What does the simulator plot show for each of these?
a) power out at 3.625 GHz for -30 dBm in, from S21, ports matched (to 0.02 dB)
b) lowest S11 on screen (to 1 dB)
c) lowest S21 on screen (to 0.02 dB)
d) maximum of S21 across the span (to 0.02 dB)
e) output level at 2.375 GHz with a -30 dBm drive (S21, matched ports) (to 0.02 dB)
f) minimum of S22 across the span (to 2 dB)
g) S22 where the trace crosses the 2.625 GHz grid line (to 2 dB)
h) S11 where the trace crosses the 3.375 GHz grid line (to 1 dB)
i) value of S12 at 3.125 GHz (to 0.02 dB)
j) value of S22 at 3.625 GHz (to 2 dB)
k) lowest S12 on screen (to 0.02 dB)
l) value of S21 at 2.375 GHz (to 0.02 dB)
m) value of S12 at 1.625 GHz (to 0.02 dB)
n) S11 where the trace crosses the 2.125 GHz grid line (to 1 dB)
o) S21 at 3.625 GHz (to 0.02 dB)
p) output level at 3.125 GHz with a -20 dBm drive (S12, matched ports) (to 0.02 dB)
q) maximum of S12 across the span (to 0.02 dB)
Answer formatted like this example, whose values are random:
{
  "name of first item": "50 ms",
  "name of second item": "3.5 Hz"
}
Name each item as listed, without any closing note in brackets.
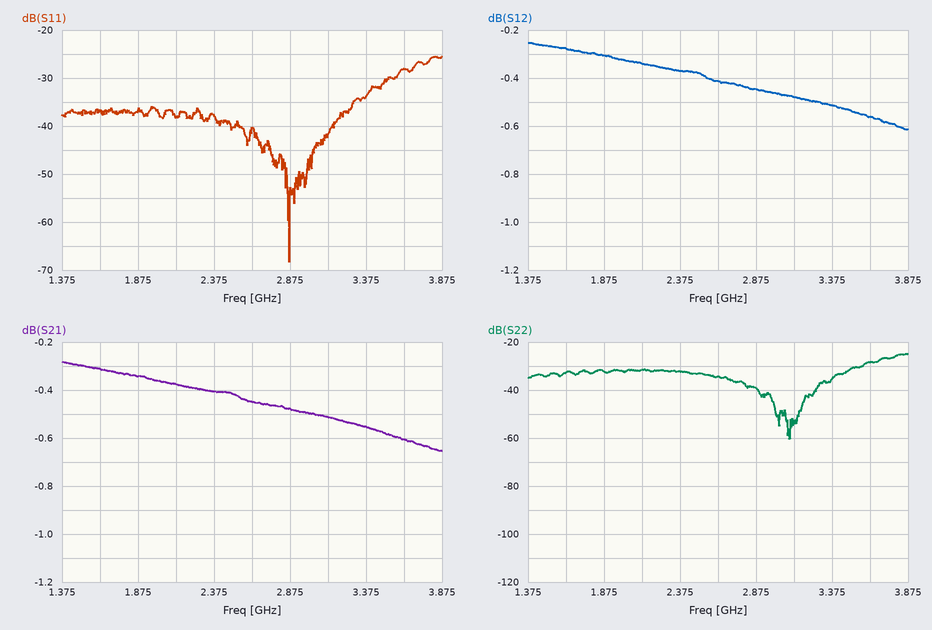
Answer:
{
  "power out at 3.625 GHz for -30 dBm in, from S21, ports matched": "-30.60 dBm",
  "lowest S11 on screen": "-68 dB",
  "lowest S21 on screen": "-0.66 dB",
  "maximum of S21 across the span": "-0.28 dB",
  "output level at 2.375 GHz with a -30 dBm drive (S21, matched ports)": "-30.40 dBm",
  "minimum of S22 across the span": "-60 dB",
  "S22 where the trace crosses the 2.625 GHz grid line": "-34 dB",
  "S11 where the trace crosses the 3.375 GHz grid line": "-34 dB",
  "value of S12 at 3.125 GHz": "-0.48 dB",
  "value of S22 at 3.625 GHz": "-28 dB",
  "lowest S12 on screen": "-0.62 dB",
  "value of S21 at 2.375 GHz": "-0.40 dB",
  "value of S12 at 1.625 GHz": "-0.28 dB",
  "S11 where the trace crosses the 2.125 GHz grid line": "-38 dB",
  "S21 at 3.625 GHz": "-0.60 dB",
  "output level at 3.125 GHz with a -20 dBm drive (S12, matched ports)": "-20.48 dBm",
  "maximum of S12 across the span": "-0.26 dB"
}
